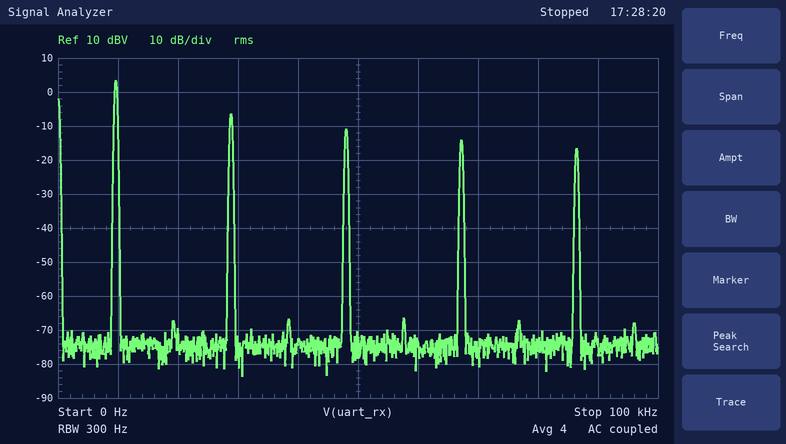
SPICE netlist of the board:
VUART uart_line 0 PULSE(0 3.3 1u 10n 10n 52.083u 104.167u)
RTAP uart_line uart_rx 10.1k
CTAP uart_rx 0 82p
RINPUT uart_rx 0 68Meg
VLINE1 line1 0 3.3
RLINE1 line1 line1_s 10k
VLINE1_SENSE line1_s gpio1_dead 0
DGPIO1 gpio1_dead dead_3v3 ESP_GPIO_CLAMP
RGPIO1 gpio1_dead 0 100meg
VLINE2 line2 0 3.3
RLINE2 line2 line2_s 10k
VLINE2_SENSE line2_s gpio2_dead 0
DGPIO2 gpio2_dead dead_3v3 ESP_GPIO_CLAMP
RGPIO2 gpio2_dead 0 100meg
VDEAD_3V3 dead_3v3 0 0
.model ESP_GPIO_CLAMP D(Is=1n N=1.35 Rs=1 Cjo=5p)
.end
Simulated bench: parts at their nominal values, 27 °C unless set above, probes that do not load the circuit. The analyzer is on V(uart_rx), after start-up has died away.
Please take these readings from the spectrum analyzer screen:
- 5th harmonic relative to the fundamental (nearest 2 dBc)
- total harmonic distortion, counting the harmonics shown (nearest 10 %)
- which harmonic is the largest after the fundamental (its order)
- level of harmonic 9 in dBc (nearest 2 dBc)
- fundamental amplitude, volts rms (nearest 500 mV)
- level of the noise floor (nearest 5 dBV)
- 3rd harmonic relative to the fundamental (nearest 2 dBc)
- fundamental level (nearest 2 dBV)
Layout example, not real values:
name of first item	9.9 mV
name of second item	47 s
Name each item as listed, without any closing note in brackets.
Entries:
5th harmonic relative to the fundamental	-14 dBc
total harmonic distortion, counting the harmonics shown	40 %
which harmonic is the largest after the fundamental	3
level of harmonic 9 in dBc	-20 dBc
fundamental amplitude, volts rms	1.5 V
level of the noise floor	-75 dBV
3rd harmonic relative to the fundamental	-10 dBc
fundamental level	4 dBV
